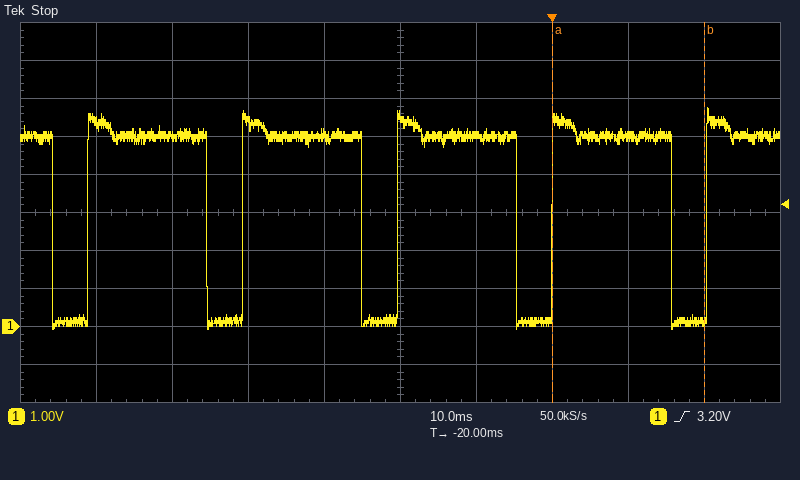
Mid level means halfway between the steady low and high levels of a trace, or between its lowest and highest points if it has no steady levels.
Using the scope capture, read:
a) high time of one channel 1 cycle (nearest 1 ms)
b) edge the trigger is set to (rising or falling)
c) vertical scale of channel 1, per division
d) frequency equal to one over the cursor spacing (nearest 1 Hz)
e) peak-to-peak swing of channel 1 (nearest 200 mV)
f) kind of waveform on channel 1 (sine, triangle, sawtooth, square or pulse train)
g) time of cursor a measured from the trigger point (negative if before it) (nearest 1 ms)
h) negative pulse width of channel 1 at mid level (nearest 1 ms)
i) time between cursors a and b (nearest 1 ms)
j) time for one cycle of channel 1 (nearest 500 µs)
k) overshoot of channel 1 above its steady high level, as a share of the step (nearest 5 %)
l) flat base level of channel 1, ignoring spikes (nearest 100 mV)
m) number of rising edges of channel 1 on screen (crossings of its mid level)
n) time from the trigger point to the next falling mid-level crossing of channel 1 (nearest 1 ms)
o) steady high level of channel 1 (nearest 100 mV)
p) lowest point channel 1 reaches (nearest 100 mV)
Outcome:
16 ms
rising
1 V
50 Hz
5.8 V
pulse train
0 ms
5 ms
20 ms
20.5 ms
15 %
100 mV
5
16 ms
5.0 V
-100 mV
